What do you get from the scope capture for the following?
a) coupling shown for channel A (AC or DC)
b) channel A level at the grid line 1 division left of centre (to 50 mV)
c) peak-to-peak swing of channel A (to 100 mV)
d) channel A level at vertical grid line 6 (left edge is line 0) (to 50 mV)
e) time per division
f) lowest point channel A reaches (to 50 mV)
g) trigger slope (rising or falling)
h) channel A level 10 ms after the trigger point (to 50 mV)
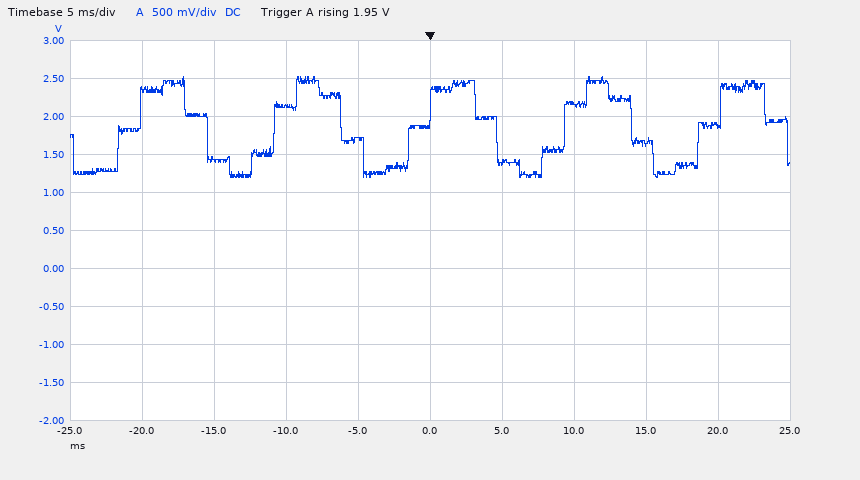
DC
1.70 V
1.30 V
1.40 V
5 ms
1.20 V
rising
2.15 V
